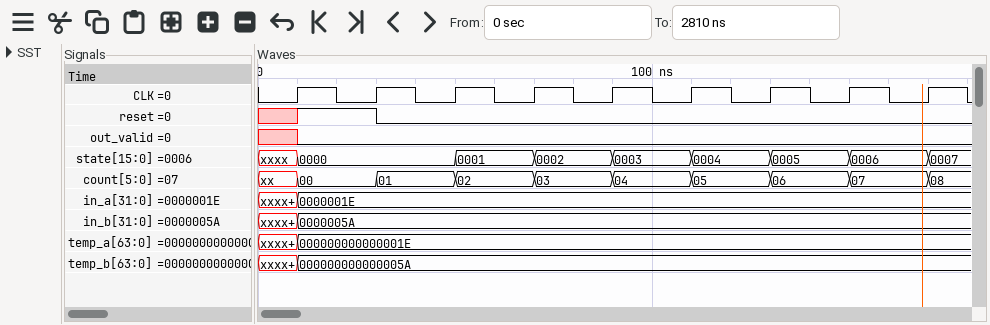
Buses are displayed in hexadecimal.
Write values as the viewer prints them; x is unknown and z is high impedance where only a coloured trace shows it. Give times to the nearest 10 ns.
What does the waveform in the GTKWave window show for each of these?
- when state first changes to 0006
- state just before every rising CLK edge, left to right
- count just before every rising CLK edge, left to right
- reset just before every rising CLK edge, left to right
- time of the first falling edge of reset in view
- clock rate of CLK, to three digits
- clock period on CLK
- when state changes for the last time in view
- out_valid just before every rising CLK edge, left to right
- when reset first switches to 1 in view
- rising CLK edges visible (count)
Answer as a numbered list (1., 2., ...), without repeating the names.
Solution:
1. 150 ns
2. xxxx, 0000, 0000, 0001, 0002, 0003, 0004, 0005, 0006
3. xx, 00, 01, 02, 03, 04, 05, 06, 07
4. x 1 0 0 0 0 0 0 0
5. 30 ns
6. 50.0 MHz
7. 20 ns
8. 170 ns
9. x 0 0 0 0 0 0 0 0
10. 10 ns
11. 9
